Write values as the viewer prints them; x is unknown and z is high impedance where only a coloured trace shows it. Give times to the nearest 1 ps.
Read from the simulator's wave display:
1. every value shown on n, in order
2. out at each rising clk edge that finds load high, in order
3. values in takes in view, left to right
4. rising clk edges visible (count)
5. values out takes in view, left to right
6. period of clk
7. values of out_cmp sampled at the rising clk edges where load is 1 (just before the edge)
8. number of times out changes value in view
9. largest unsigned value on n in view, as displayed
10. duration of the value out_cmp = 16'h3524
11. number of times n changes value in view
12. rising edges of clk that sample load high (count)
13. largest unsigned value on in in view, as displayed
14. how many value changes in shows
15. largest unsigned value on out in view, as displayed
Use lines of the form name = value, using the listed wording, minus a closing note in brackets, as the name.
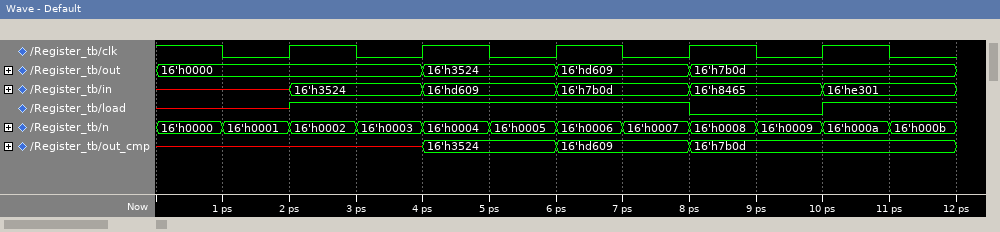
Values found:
every value shown on n, in order = 16'h0000, 16'h0001, 16'h0002, 16'h0003, 16'h0004, 16'h0005, 16'h0006, 16'h0007, 16'h0008, 16'h0009, 16'h000a, 16'h000b
out at each rising clk edge that finds load high, in order = 16'h0000, 16'h3524, 16'hd609
values in takes in view, left to right = x, 16'h3524, 16'hd609, 16'h7b0d, 16'h8465, 16'he301
rising clk edges visible = 5
values out takes in view, left to right = 16'h0000, 16'h3524, 16'hd609, 16'h7b0d
period of clk = 2 ps
values of out_cmp sampled at the rising clk edges where load is 1 = x, 16'h3524, 16'hd609
number of times out changes value in view = 3
largest unsigned value on n in view, as displayed = 16'h000b
duration of the value out_cmp = 16'h3524 = 2 ps
number of times n changes value in view = 11
rising edges of clk that sample load high = 3
largest unsigned value on in in view, as displayed = 16'he301
how many value changes in shows = 5
largest unsigned value on out in view, as displayed = 16'hd609
